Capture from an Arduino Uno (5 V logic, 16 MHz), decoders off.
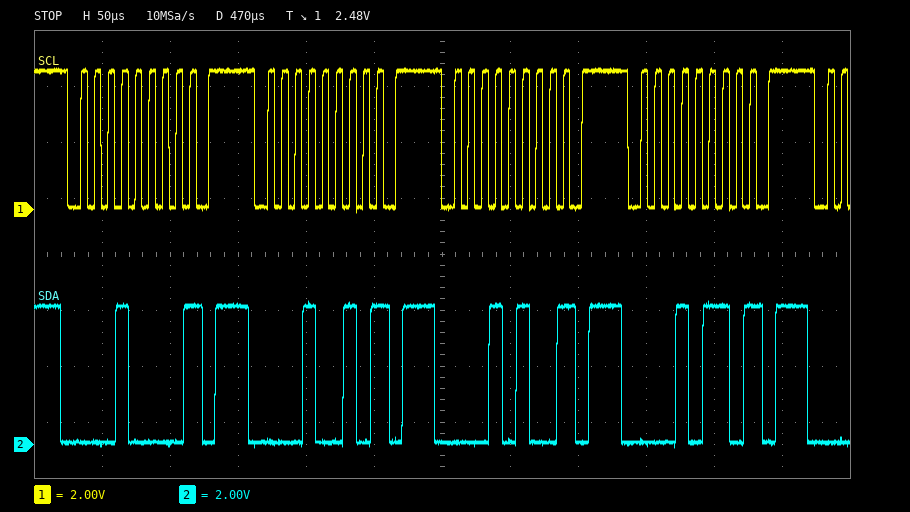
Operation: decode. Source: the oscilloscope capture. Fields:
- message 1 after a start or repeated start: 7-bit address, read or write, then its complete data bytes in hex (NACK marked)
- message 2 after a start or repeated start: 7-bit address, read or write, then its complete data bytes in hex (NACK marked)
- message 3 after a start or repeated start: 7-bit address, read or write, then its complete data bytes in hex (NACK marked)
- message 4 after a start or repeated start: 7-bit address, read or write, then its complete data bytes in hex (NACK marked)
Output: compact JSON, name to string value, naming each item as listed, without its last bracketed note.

{"message 1 after a start or repeated start: 7-bit address, read or write, then its complete data bytes in hex": "0x08 write NACK", "message 2 after a start or repeated start: 7-bit address, read or write, then its complete data bytes in hex": "0x09 write NACK", "message 3 after a start or repeated start: 7-bit address, read or write, then its complete data bytes in hex": "0x0A write NACK", "message 4 after a start or repeated start: 7-bit address, read or write, then its complete data bytes in hex": "0x0B write NACK"}
